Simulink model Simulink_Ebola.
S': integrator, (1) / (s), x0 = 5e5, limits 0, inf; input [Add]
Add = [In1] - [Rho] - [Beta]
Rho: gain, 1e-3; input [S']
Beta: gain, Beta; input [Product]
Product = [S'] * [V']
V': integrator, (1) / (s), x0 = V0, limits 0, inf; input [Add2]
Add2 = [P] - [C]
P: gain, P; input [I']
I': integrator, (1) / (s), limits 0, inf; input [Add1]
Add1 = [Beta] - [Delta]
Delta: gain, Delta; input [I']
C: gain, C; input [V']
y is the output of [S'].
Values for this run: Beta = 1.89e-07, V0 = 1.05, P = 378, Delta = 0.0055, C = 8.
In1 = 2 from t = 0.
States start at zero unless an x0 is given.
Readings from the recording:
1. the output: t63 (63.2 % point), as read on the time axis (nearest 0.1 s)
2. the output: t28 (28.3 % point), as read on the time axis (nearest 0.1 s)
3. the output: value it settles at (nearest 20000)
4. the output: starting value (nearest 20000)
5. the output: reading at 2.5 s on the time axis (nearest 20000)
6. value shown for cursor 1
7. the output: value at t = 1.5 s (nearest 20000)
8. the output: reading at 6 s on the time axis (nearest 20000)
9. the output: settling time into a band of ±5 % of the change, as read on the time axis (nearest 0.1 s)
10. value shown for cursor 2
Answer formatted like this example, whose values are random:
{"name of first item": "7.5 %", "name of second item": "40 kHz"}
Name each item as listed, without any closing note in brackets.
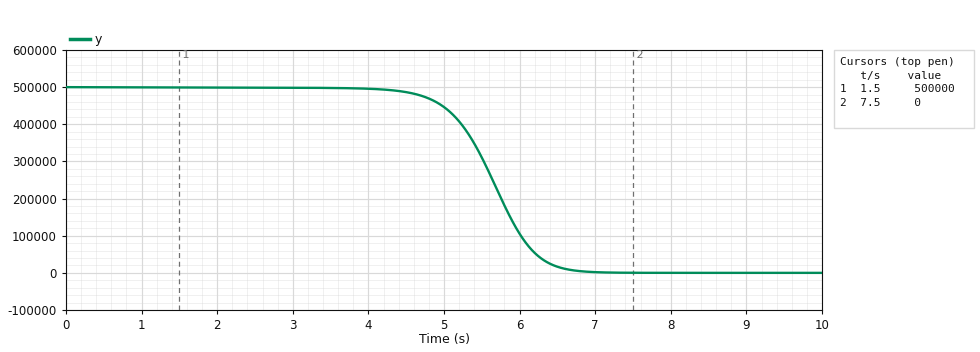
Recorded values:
{"the output: t63 (63.2 % point), as read on the time axis": "5.8 s", "the output: t28 (28.3 % point), as read on the time axis": "5.4 s", "the output: value it settles at": "0", "the output: starting value": "500000", "the output: reading at 2.5 s on the time axis": "500000", "value shown for cursor 1": "500000", "the output: value at t = 1.5 s": "500000", "the output: reading at 6 s on the time axis": "100000", "the output: settling time into a band of ±5 % of the change, as read on the time axis": "6.4 s", "value shown for cursor 2": "0"}
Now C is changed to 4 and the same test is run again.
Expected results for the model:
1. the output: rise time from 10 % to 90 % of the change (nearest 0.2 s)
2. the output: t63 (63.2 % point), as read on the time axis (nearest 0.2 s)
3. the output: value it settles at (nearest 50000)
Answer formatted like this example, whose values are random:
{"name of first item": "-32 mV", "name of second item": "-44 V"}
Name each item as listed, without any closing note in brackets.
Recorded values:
{"the output: rise time from 10 % to 90 % of the change": "0.8 s", "the output: t63 (63.2 % point), as read on the time axis": "4.2 s", "the output: value it settles at": "0"}
